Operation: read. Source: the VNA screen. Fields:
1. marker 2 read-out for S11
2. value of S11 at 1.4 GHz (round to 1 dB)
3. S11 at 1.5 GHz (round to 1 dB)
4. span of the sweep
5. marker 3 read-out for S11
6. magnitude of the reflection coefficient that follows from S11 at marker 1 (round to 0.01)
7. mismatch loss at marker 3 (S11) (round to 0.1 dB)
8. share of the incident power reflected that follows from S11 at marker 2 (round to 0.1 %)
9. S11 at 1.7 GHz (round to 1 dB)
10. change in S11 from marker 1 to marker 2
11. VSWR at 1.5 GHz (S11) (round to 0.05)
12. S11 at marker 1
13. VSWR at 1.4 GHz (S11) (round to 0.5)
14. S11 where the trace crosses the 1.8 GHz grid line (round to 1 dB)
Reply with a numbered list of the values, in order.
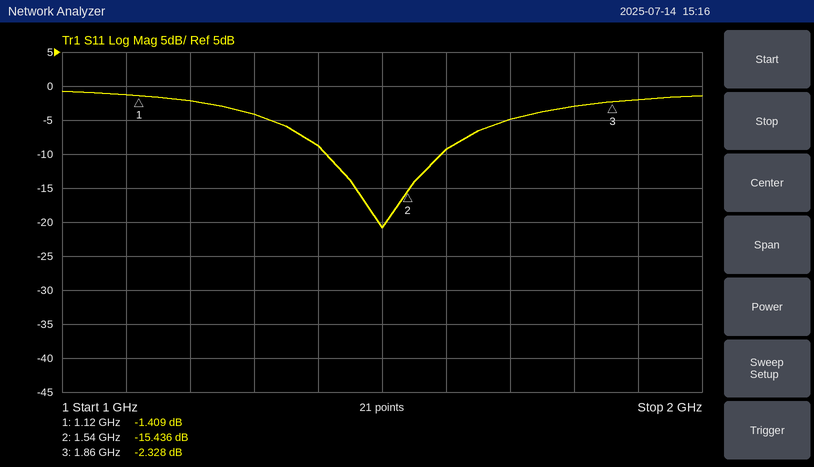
1. -15.436 dB
2. -9 dB
3. -21 dB
4. 1 GHz
5. -2.328 dB
6. 0.85
7. 3.8 dB
8. 2.9 %
9. -5 dB
10. -14.027 dB
11. 1.20
12. -1.409 dB
13. 2.0
14. -3 dB
